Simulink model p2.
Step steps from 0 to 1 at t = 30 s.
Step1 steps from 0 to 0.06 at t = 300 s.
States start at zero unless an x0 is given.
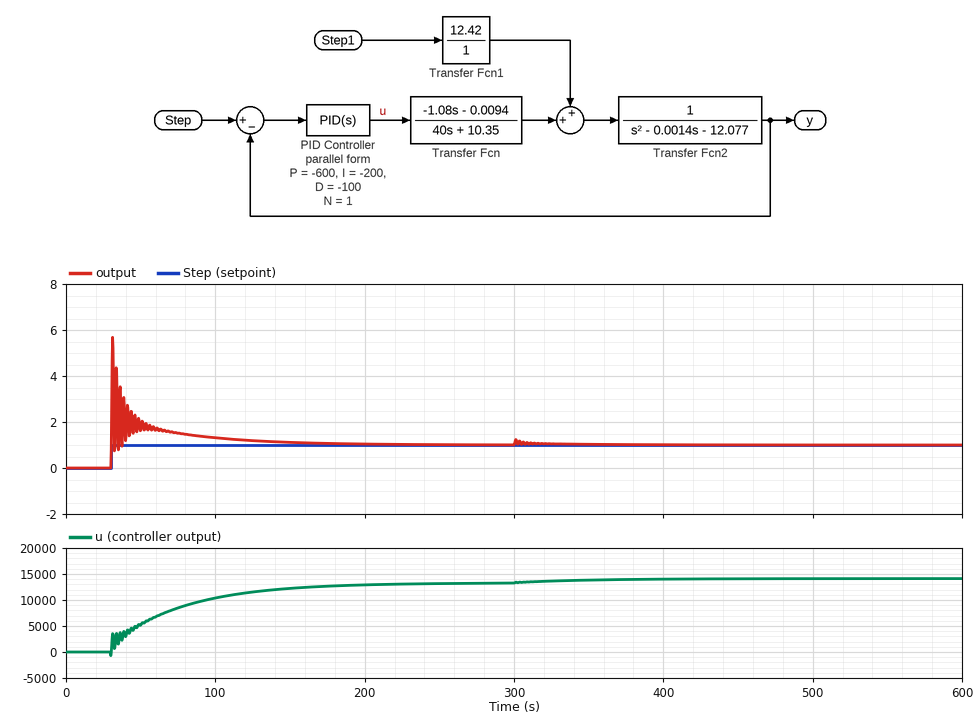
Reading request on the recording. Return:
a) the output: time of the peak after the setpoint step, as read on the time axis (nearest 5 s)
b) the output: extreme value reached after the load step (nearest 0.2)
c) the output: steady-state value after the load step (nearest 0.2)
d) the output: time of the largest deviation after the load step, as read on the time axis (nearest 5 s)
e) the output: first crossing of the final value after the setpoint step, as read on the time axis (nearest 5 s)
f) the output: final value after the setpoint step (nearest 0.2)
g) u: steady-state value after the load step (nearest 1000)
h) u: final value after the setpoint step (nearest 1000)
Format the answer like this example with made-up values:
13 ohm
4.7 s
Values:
30 s
1.2
1.0
300 s
30 s
1.0
14000
13000
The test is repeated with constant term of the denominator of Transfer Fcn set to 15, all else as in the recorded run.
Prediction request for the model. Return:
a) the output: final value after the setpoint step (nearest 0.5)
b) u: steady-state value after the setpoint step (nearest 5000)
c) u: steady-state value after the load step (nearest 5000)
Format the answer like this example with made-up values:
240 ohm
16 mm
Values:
1.0
20000
20000
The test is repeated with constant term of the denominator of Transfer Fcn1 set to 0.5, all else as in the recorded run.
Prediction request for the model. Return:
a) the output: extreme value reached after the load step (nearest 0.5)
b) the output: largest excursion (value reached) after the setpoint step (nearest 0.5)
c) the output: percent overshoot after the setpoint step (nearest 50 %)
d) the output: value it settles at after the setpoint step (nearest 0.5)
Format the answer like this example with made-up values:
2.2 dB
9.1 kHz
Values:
1.5
5.5
450 %
1.0
